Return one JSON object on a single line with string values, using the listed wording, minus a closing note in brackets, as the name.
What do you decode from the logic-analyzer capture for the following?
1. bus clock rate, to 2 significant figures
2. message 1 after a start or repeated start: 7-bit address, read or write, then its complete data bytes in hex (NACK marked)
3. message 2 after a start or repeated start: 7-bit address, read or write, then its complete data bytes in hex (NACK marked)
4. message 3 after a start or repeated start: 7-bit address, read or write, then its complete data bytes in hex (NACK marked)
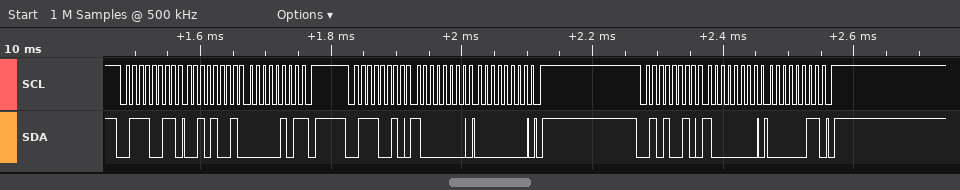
{"bus clock rate, to 2 significant figures": "100 kHz", "message 1 after a start or repeated start: 7-bit address, read or write, then its complete data bytes in hex": "0x39 read: 29 05 NACK", "message 2 after a start or repeated start: 7-bit address, read or write, then its complete data bytes in hex": "0x39 write: 80 00", "message 3 after a start or repeated start: 7-bit address, read or write, then its complete data bytes in hex": "0x29 write: 80 03"}
